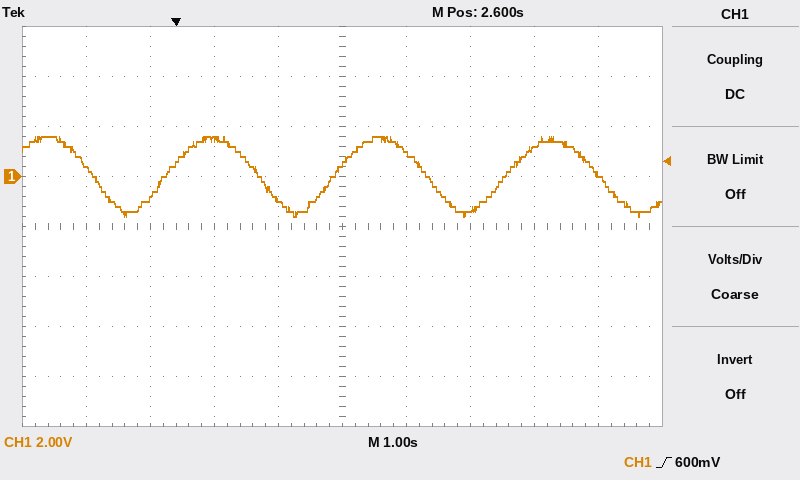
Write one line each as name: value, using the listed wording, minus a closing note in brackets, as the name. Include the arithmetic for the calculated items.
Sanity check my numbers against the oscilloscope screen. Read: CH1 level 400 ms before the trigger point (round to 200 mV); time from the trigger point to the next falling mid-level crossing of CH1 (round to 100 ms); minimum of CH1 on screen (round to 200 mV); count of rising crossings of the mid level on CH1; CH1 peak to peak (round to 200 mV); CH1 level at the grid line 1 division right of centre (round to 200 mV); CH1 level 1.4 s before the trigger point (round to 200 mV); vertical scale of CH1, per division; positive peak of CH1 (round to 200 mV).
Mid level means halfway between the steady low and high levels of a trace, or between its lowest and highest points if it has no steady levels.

CH1 level 400 ms before the trigger point: -800 mV
time from the trigger point to the next falling mid-level crossing of CH1: 1.3 s
minimum of CH1 on screen: -1.6 V
count of rising crossings of the mid level on CH1: 3
CH1 peak to peak: 1.6 V − (-1.6 V) = 3.2 V
CH1 level at the grid line 1 division right of centre: 1.0 V
CH1 level 1.4 s before the trigger point: 400 mV
vertical scale of CH1, per division: 2 V
positive peak of CH1: 1.6 V
